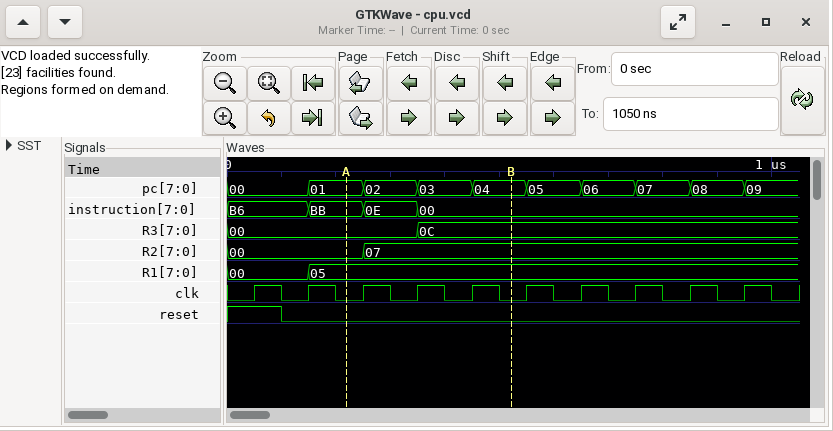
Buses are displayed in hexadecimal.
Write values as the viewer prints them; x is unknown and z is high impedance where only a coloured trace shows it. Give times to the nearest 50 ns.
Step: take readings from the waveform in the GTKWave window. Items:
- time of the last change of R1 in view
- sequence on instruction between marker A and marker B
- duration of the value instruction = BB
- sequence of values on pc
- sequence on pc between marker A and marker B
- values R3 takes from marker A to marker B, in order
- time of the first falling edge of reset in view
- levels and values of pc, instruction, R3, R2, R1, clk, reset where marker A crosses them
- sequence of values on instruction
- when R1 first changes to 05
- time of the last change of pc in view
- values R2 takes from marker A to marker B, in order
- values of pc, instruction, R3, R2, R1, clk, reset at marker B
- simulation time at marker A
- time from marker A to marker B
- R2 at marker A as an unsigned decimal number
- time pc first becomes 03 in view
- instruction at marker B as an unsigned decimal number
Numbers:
150 ns
BB, 0E, 00
100 ns
00, 01, 02, 03, 04, 05, 06, 07, 08, 09
01, 02, 03, 04
00, 0C
100 ns
pc=01, instruction=BB, R3=00, R2=00, R1=05, clk=0, reset=0
B6, BB, 0E, 00
150 ns
950 ns
00, 07
pc=04, instruction=00, R3=0C, R2=07, R1=05, clk=0, reset=0
200 ns
300 ns
0
350 ns
0
